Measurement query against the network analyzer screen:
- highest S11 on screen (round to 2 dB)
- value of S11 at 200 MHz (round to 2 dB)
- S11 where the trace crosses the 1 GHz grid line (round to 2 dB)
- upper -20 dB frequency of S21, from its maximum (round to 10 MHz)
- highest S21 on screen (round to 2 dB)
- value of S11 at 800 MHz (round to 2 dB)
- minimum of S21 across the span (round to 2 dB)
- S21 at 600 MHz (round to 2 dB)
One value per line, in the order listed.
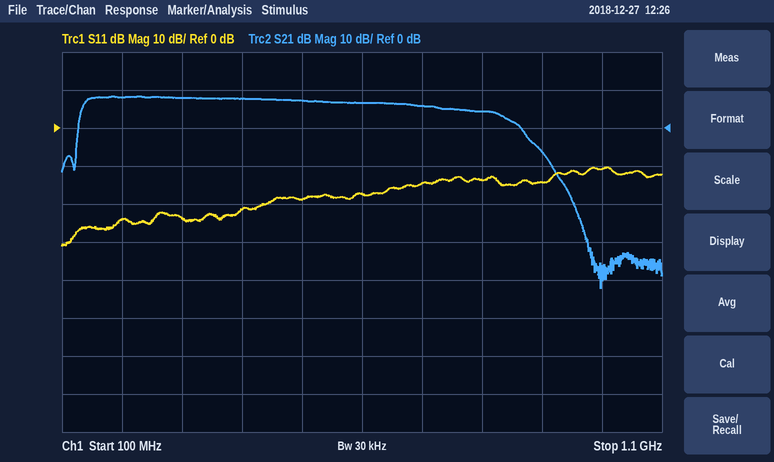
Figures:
-10 dB
-24 dB
-10 dB
920 MHz
8 dB
-14 dB
-42 dB
6 dB
